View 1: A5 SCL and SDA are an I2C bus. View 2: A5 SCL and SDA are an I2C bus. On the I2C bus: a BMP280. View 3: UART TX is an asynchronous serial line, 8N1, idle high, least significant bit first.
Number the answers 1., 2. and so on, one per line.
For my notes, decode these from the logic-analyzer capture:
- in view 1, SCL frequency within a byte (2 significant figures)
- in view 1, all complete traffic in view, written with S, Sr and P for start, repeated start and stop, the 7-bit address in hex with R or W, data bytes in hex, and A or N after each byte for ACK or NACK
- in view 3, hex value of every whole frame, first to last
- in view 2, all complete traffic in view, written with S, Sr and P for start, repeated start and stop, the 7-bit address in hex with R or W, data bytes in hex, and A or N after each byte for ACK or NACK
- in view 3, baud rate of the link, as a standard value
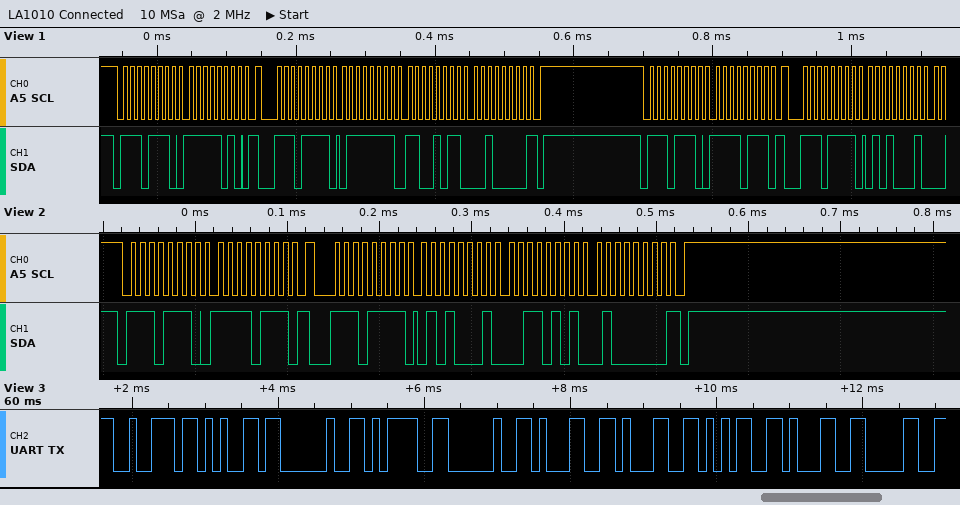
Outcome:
1. 100 kHz
2. S 77W A FA A Sr 77R A 7F A CB A 20 N P S 77W A F7 A Sr 77R A 51 A
3. 72 65 20 3D 20 31 31 35 31 30
4. S 77W A F7 A Sr 77R A 51 A 35 A 40 N P
5. 9600 baud
